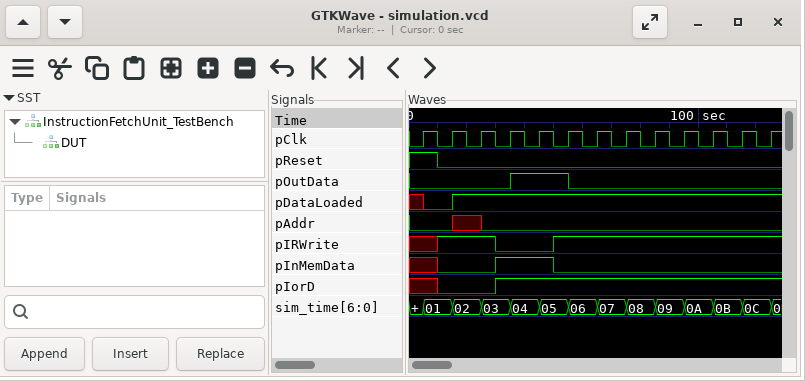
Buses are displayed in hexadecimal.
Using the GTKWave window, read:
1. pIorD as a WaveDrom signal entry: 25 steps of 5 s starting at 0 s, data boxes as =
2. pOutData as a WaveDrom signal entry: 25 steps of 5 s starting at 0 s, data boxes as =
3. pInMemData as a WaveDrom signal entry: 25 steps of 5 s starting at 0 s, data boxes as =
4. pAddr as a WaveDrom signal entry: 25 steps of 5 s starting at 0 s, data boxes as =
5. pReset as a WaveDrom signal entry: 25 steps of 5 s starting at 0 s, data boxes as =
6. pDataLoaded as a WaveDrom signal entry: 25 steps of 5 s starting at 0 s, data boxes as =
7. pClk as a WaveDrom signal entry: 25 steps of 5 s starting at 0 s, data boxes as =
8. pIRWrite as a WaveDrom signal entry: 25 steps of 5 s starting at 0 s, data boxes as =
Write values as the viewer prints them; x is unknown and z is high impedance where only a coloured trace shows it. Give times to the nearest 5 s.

{name: 'pIorD', wave: 'x.0...1..................'}
{name: 'pOutData', wave: '0......1...0.............'}
{name: 'pInMemData', wave: 'x.0...1...0..............'}
{name: 'pAddr', wave: '0..x.0...................'}
{name: 'pReset', wave: '1.0......................'}
{name: 'pDataLoaded', wave: 'x0.1.....................'}
{name: 'pClk', wave: '0101010101010101010101010'}
{name: 'pIRWrite', wave: 'x.1...0...1..............'}
